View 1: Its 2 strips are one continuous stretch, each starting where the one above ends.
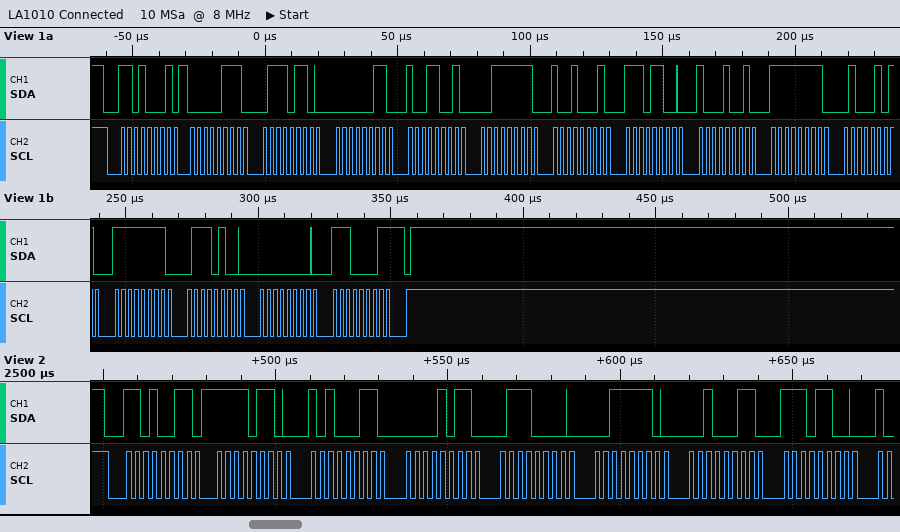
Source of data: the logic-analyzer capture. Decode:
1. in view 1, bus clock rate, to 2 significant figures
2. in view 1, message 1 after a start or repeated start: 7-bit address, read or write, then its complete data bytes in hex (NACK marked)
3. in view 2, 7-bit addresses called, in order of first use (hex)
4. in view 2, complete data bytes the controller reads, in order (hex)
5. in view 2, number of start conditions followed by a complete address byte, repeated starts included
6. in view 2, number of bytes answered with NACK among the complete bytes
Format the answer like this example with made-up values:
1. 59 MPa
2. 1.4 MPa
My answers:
1. 400 kHz
2. 0x68 read: 07 76 03 99 3F 91 EC 89 FF 45 FF 74 00 E1 NACK
3. 0x69
4. F6 A3 0B 70 3E 23 EC
5. 1
6. 0
